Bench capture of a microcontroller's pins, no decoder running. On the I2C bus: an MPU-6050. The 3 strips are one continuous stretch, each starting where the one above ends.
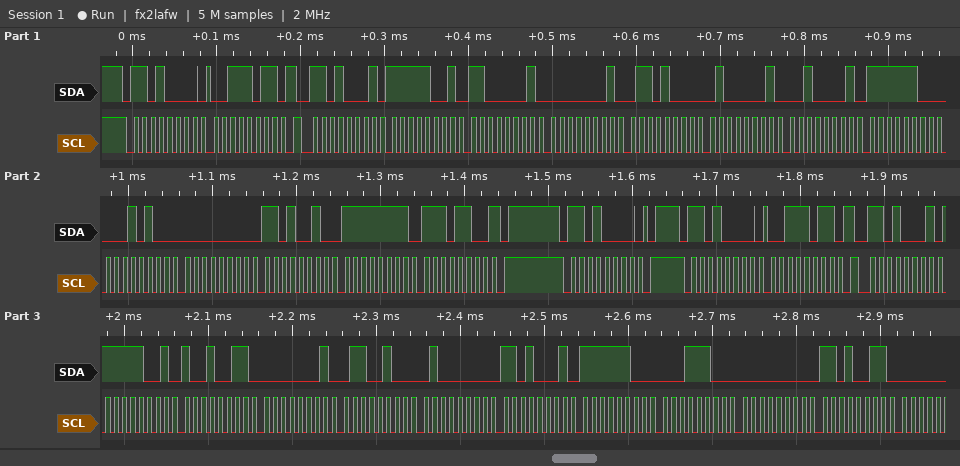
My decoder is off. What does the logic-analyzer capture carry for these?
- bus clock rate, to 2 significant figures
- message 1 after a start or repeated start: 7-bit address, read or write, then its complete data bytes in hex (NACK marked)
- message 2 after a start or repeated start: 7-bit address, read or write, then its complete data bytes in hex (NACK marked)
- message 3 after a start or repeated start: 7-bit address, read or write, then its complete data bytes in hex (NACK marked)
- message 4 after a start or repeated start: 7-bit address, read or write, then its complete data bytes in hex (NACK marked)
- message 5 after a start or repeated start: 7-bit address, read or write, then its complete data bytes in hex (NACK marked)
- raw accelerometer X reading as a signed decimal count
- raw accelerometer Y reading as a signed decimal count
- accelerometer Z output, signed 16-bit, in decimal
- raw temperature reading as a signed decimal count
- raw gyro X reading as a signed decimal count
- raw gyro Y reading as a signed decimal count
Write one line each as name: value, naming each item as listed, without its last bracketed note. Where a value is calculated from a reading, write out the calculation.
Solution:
bus clock rate, to 2 significant figures: 100 kHz
message 1 after a start or repeated start: 7-bit address, read or write, then its complete data bytes in hex: 0x68 write: 3B
message 2 after a start or repeated start: 7-bit address, read or write, then its complete data bytes in hex: 0x68 read: F9 C1 01 68 41 21 FC 14 00 D2 FF EC NACK
message 3 after a start or repeated start: 7-bit address, read or write, then its complete data bytes in hex: 0x68 write
message 4 after a start or repeated start: 7-bit address, read or write, then its complete data bytes in hex: 0x68 write: 3B
message 5 after a start or repeated start: 7-bit address, read or write, then its complete data bytes in hex: 0x68 read: F9 93 01 64 40 D1 FC 1C 00 D3
raw accelerometer X reading as a signed decimal count: 0xF9C1 = -1599
raw accelerometer Y reading as a signed decimal count: 0x0168 = 360
accelerometer Z output, signed 16-bit, in decimal: 0x4121 = 16673
raw temperature reading as a signed decimal count: 0xFC14 = -1004
raw gyro X reading as a signed decimal count: 0x00D2 = 210
raw gyro Y reading as a signed decimal count: 0xFFEC = -20
